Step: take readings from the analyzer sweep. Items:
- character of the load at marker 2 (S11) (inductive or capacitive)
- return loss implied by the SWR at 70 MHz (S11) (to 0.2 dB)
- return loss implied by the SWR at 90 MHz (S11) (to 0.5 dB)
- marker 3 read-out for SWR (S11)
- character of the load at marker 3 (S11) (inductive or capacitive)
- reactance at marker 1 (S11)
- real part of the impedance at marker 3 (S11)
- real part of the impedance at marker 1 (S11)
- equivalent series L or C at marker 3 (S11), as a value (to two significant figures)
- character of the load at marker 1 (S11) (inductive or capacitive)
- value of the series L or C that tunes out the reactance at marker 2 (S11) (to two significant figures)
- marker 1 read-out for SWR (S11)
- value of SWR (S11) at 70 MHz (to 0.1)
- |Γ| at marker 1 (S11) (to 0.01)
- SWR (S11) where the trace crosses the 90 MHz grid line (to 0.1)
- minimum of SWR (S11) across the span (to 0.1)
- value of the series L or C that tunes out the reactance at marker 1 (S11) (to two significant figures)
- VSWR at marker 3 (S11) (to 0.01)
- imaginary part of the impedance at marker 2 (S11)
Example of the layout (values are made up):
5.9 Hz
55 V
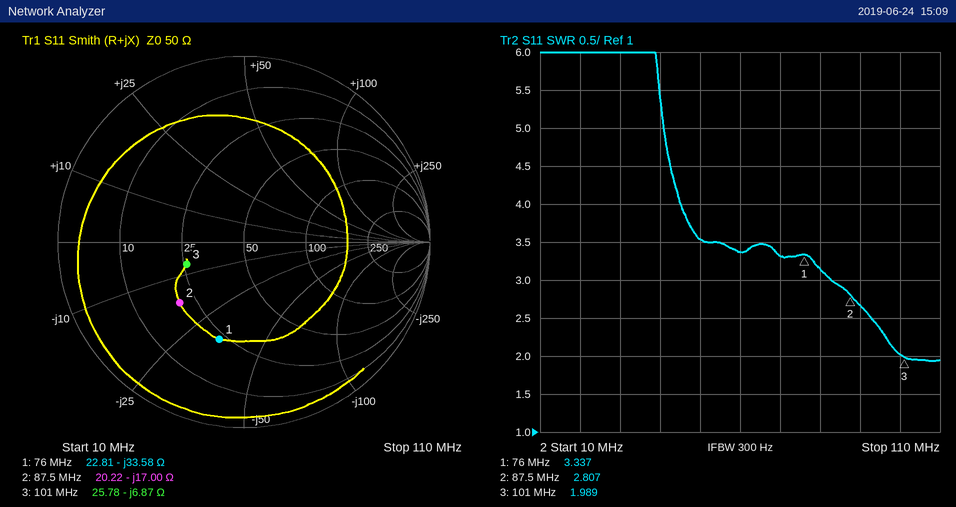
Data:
capacitive
5.4 dB
7.0 dB
1.989
capacitive
-33.58 Ω
25.78 Ω
22.81 Ω
230 pF
capacitive
31 nH
3.337
3.3
0.54
2.7
1.9
70 nH
1.99
-17.00 Ω
